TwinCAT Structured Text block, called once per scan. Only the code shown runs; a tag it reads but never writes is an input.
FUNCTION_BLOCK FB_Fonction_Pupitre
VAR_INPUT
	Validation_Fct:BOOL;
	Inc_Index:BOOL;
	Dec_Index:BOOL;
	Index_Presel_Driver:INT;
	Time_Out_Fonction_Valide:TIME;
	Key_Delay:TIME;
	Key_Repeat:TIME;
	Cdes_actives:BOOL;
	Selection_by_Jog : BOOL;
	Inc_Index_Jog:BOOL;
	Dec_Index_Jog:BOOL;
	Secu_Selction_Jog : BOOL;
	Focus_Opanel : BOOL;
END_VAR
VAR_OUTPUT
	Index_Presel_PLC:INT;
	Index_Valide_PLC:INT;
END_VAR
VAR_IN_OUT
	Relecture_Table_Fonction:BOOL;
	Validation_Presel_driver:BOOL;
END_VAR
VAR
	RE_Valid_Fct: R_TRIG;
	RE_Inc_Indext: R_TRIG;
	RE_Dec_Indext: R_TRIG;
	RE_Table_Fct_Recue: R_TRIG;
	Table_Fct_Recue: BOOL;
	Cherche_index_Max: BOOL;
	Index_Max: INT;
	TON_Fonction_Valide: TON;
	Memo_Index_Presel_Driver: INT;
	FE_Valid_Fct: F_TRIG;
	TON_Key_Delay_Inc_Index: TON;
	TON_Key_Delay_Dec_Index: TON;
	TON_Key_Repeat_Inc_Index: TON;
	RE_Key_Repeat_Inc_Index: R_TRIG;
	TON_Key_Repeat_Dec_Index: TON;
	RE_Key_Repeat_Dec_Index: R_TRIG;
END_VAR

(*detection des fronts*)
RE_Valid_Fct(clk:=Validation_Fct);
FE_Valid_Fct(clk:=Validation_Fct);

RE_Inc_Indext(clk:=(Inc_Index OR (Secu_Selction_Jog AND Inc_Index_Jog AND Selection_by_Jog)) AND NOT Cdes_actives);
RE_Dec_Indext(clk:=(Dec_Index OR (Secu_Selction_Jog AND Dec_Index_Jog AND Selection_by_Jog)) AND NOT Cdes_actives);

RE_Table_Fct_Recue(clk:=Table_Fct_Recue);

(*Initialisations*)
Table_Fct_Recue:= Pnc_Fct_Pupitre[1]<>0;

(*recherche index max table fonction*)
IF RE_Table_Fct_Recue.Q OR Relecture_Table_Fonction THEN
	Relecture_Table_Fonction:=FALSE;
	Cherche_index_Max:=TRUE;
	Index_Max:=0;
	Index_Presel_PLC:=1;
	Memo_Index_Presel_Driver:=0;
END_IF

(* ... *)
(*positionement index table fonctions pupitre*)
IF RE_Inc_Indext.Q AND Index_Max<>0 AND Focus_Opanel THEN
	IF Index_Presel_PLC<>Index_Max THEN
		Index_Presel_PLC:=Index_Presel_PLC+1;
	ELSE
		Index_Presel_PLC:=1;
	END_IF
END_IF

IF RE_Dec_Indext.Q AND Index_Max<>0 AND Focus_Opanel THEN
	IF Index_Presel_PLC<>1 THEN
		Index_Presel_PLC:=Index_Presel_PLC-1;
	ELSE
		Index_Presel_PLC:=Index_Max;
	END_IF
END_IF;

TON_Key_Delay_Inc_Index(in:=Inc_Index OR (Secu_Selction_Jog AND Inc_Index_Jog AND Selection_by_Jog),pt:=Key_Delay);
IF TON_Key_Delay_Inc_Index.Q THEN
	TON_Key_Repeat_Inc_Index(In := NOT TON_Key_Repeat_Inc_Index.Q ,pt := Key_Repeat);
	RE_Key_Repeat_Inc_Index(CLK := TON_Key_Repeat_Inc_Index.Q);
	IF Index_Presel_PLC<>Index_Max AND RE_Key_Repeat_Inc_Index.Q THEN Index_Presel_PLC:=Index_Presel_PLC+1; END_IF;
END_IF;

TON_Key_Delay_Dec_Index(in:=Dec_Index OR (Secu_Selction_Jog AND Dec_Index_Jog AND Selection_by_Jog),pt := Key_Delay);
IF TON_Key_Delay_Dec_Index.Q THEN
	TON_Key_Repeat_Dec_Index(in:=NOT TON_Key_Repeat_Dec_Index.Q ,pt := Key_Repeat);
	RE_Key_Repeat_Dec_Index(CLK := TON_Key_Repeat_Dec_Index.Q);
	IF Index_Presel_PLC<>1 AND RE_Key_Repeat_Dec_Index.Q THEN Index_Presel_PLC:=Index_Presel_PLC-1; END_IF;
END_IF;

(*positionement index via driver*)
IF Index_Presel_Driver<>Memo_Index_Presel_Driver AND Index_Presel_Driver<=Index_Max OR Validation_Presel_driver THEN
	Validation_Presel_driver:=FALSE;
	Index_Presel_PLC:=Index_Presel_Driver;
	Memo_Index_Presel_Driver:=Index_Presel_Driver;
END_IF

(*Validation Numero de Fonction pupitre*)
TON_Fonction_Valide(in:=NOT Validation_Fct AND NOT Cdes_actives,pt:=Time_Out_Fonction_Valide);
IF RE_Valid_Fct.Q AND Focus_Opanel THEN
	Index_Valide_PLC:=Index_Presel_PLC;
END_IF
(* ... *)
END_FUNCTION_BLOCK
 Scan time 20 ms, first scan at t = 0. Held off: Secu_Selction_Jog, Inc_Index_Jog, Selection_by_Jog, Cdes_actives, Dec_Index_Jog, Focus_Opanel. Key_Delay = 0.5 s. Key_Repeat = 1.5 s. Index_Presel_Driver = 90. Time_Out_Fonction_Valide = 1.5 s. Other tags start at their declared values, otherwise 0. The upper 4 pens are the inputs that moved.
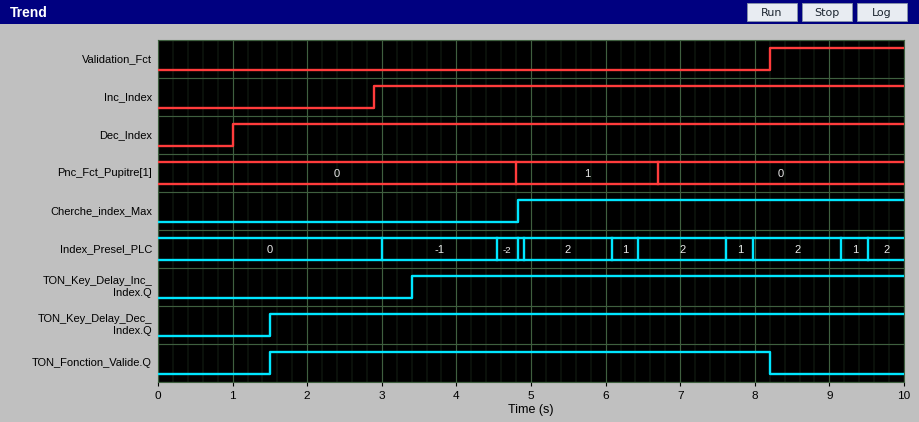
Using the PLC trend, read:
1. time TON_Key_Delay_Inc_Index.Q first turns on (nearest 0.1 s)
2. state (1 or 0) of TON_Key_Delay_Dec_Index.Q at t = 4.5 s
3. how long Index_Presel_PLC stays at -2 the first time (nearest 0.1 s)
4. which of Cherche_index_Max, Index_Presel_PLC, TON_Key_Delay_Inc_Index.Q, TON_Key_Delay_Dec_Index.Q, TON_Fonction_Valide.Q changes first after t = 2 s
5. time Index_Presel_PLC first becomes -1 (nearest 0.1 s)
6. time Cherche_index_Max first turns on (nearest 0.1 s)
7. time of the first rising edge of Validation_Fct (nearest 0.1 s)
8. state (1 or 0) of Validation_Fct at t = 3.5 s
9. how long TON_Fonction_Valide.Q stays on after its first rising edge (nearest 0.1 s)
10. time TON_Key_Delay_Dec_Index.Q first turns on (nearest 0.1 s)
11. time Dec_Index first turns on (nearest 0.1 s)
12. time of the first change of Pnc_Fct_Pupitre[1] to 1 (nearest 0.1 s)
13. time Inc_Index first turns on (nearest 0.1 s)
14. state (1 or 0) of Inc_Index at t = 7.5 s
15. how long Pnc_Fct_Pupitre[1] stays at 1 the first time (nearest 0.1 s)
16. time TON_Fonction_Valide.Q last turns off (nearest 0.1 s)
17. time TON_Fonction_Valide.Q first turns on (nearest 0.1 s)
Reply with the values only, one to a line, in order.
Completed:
3.4 s
1
0.3 s
Index_Presel_PLC
3.0 s
4.8 s
8.2 s
0
6.7 s
1.5 s
1.0 s
4.8 s
2.9 s
1
1.9 s
8.2 s
1.5 s
